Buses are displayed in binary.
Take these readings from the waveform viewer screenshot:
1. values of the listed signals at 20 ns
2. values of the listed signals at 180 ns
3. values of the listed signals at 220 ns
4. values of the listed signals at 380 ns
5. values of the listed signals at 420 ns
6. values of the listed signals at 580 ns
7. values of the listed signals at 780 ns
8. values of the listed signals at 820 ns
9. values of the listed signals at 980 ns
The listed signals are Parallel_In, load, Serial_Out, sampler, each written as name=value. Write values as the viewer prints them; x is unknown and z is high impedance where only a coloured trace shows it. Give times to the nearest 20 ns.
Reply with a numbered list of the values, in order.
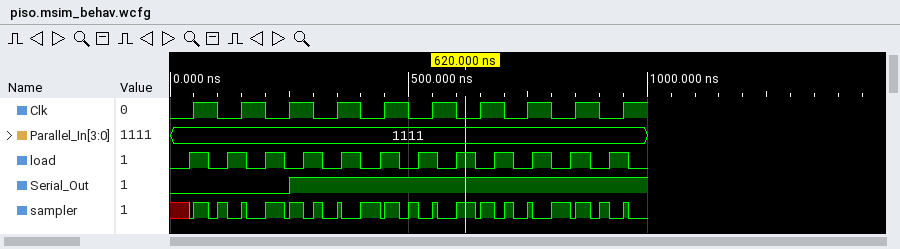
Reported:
1. Parallel_In=1111, load=0, Serial_Out=0, sampler=x
2. Parallel_In=1111, load=0, Serial_Out=0, sampler=0
3. Parallel_In=1111, load=1, Serial_Out=0, sampler=1
4. Parallel_In=1111, load=1, Serial_Out=1, sampler=0
5. Parallel_In=1111, load=0, Serial_Out=1, sampler=1
6. Parallel_In=1111, load=0, Serial_Out=1, sampler=0
7. Parallel_In=1111, load=1, Serial_Out=1, sampler=0
8. Parallel_In=1111, load=0, Serial_Out=1, sampler=1
9. Parallel_In=1111, load=0, Serial_Out=1, sampler=0
